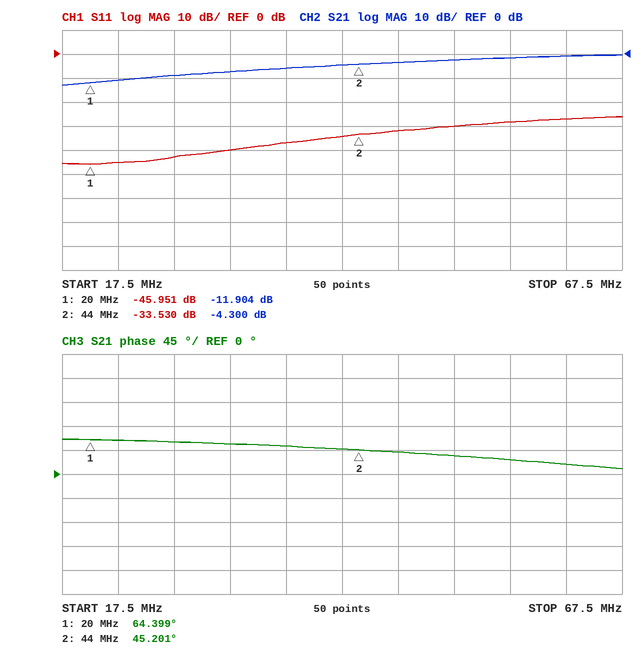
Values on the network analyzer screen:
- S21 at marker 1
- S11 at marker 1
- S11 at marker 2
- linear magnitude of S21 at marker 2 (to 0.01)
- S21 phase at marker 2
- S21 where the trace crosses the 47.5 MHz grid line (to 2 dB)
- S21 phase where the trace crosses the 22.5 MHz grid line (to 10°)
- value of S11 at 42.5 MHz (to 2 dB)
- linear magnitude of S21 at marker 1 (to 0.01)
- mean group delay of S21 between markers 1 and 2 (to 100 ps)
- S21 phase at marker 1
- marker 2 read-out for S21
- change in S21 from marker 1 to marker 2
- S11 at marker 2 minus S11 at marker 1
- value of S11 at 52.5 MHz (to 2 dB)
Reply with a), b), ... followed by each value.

a) -11.904 dB
b) -45.951 dB
c) -33.530 dB
d) 0.61
e) 45.201°
f) -4 dB
g) 60°
h) -34 dB
i) 0.25
j) 2.2 ns
k) 64.399°
l) -4.300 dB
m) 7.604 dB
n) 12.421 dB
o) -30 dB
